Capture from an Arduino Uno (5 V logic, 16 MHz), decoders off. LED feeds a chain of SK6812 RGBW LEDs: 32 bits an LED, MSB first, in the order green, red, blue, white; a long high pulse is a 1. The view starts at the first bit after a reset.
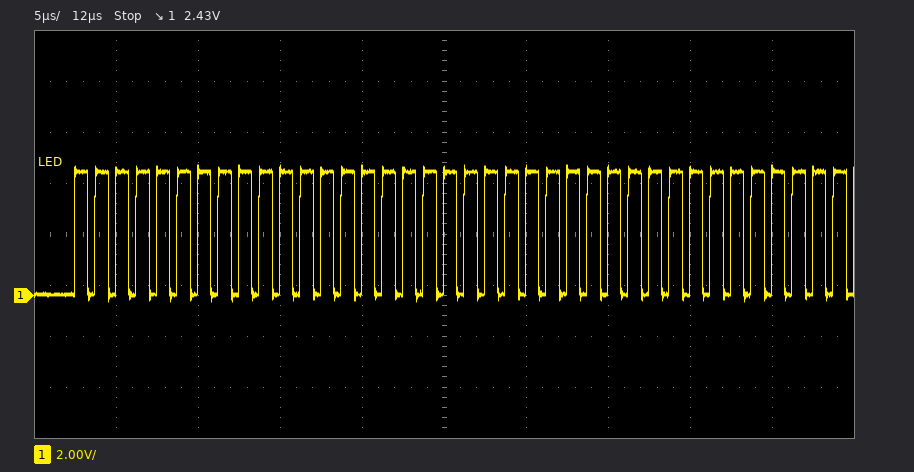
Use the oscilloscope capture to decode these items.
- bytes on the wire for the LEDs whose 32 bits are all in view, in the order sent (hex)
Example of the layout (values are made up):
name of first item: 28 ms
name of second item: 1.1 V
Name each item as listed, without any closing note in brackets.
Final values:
bytes on the wire for the LEDs whose 32 bits are all in view, in the order sent: FF FF FF FF
